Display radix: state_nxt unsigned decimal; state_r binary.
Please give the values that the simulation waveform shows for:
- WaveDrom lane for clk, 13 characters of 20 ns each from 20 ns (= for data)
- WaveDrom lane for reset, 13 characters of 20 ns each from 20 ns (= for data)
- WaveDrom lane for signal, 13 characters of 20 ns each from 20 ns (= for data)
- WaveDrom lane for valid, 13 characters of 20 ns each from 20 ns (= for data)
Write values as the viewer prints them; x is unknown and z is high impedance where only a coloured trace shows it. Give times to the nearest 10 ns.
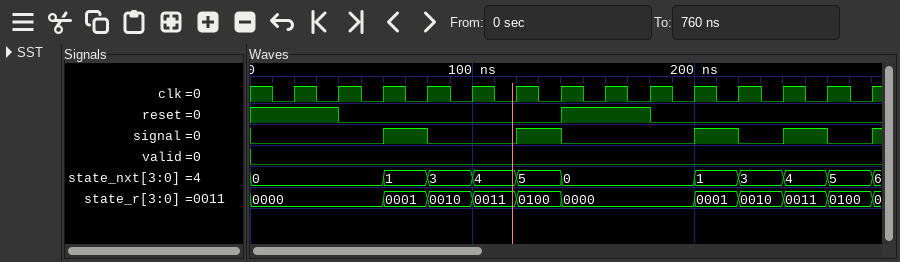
{name: 'clk', wave: 'p............'}
{name: 'reset', wave: '10....1.0....'}
{name: 'signal', wave: '0.10.10..1010'}
{name: 'valid', wave: '0............'}
